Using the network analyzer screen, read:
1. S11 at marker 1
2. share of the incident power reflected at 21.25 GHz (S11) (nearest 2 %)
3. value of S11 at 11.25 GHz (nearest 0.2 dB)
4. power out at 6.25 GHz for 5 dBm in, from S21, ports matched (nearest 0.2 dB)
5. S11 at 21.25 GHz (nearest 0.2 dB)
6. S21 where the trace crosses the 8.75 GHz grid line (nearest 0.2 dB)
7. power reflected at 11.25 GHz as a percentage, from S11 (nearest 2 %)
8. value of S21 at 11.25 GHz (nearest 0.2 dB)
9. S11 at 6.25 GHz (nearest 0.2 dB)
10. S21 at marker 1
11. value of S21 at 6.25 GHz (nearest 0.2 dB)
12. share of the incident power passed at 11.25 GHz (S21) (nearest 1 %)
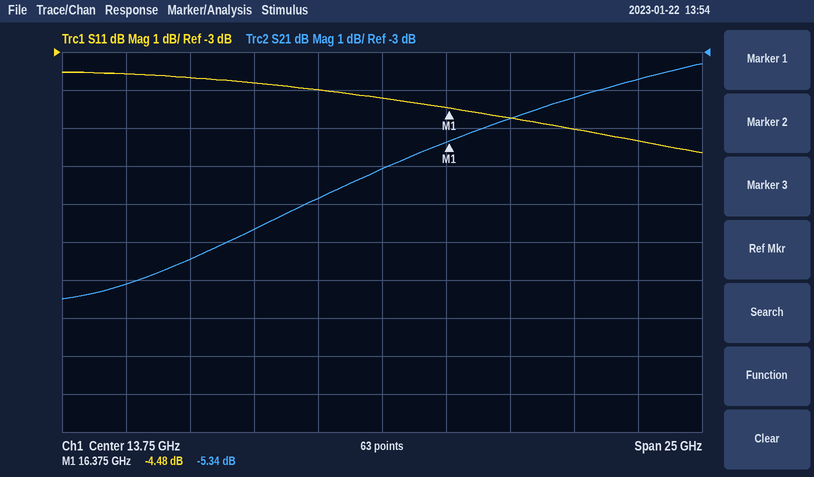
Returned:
-4.48 dB
32 %
-4.0 dB
-3.4 dBm
-5.0 dB
-7.6 dB
40 %
-6.8 dB
-3.6 dB
-5.34 dB
-8.4 dB
21 %
